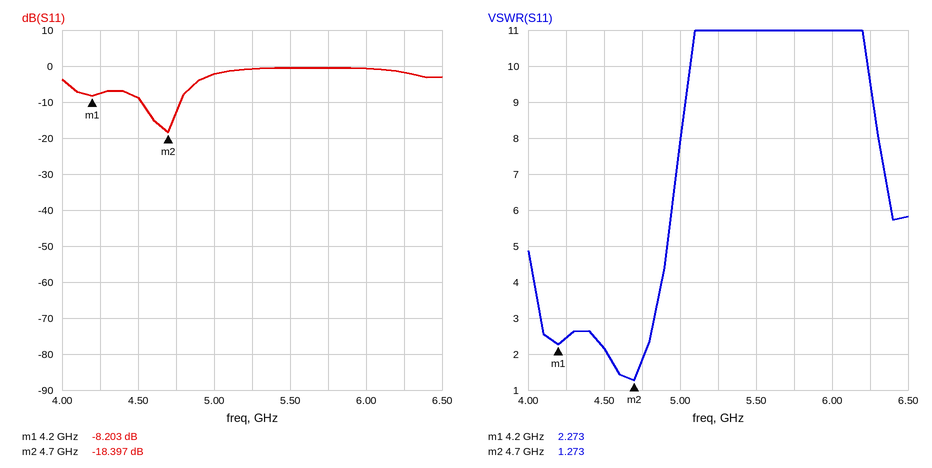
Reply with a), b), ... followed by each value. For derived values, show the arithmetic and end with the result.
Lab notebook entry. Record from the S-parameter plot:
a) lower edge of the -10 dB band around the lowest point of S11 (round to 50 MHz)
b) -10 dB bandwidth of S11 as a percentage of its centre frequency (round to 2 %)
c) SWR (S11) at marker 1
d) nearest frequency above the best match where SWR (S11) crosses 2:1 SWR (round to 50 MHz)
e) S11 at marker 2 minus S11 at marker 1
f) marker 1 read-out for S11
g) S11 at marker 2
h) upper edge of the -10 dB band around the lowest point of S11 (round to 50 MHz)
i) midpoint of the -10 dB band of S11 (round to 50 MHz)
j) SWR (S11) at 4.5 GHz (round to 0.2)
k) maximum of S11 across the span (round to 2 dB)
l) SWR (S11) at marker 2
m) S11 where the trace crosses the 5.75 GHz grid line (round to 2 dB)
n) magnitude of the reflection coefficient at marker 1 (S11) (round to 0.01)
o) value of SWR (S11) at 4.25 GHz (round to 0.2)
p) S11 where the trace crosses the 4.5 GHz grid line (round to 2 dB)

a) 4.50 GHz
b) 300 MHz / 4.65 GHz ≈ 6 %
c) 2.273
d) 4.75 GHz
e) -18.397 − (-8.203) = -10.194 dB
f) -8.203 dB
g) -18.397 dB
h) 4.80 GHz
i) 4.65 GHz
j) 2.2
k) 0 dB
l) 1.273
m) 0 dB
n) 10^(-8.203/20) ≈ 0.39
o) 2.4
p) -8 dB
